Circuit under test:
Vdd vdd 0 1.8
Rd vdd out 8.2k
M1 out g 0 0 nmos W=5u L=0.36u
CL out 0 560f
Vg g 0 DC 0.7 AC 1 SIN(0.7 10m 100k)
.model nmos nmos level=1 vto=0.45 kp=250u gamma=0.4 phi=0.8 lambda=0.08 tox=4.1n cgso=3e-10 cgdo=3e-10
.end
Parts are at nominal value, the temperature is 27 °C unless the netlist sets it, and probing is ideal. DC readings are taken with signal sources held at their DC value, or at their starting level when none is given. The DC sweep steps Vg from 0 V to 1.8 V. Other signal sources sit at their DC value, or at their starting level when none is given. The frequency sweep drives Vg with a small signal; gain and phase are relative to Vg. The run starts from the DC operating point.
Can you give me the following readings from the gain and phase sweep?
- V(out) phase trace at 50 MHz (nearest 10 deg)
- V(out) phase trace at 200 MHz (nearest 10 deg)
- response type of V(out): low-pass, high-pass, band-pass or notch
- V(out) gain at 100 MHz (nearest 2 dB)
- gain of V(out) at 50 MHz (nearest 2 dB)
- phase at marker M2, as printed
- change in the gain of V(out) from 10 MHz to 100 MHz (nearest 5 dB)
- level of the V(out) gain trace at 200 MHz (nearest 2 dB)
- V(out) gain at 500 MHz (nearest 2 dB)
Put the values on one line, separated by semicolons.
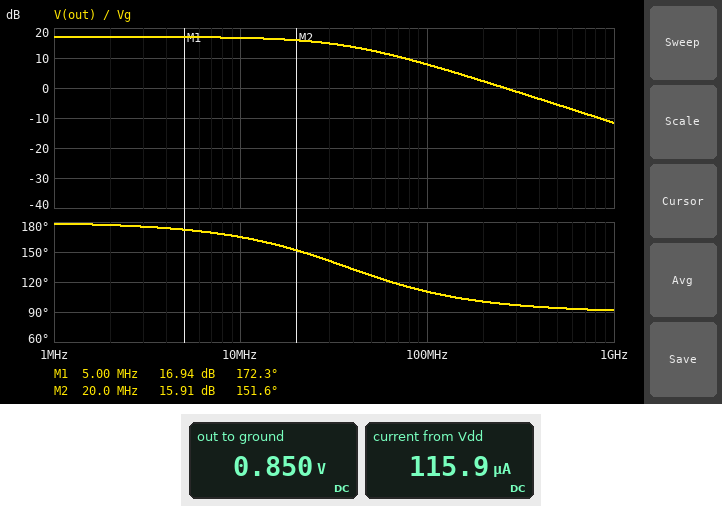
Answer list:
130 deg; 100 deg; low-pass; 8 dB; 12 dB; 151.6 deg; -10 dB; 2 dB; -6 dB
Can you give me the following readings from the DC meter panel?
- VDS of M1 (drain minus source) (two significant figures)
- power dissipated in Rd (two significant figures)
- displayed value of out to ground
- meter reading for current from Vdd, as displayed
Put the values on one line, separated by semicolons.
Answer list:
850 mV; 110 µW; 0.850 V; 115.9 µA
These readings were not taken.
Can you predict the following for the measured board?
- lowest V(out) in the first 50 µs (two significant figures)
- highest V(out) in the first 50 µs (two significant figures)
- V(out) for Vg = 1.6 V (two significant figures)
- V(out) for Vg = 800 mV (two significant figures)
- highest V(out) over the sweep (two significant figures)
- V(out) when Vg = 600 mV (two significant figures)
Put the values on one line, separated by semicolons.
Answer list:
780 mV; 920 mV; 54 mV; 230 mV; 1.8 V; 1.4 V
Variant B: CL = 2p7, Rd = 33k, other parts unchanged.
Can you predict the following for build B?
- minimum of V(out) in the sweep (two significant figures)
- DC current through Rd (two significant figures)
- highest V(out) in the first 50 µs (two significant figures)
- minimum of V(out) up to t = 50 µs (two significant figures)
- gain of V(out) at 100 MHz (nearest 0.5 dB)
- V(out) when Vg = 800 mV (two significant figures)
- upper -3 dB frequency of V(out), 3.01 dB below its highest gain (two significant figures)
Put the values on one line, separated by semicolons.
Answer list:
12 mV; 52 µA; 74 mV; 66 mV; -17.5 dB; 47 mV; 39 MHz
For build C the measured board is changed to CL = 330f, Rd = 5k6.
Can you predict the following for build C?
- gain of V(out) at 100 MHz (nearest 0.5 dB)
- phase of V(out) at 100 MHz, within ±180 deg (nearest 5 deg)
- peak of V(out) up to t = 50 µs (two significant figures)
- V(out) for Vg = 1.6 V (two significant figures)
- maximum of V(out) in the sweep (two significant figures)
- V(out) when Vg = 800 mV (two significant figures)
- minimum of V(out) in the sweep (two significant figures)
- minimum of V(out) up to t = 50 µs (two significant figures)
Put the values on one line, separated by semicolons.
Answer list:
10.5 dB; 130 deg; 1.2 V; 79 mV; 1.8 V; 560 mV; 67 mV; 1.1 V
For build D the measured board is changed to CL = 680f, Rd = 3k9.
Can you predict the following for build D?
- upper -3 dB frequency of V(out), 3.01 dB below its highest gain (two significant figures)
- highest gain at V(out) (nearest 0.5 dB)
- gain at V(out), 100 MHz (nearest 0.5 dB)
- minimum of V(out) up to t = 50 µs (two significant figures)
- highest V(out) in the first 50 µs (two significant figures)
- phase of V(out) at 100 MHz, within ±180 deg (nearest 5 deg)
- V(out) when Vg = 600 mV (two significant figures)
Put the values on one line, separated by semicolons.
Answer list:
62 MHz; 11.0 dB; 5.5 dB; 1.3 V; 1.4 V; 120 deg; 1.6 V
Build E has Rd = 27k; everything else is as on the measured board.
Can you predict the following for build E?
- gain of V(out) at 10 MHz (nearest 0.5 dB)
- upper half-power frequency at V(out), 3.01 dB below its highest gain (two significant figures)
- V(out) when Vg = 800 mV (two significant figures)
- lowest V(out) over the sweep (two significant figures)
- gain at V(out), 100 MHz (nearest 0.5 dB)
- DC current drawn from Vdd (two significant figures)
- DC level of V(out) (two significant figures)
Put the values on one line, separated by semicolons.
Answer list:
-6.0 dB; 170 MHz; 58 mV; 14 mV; -7.0 dB; 63 µA; 88 mV
